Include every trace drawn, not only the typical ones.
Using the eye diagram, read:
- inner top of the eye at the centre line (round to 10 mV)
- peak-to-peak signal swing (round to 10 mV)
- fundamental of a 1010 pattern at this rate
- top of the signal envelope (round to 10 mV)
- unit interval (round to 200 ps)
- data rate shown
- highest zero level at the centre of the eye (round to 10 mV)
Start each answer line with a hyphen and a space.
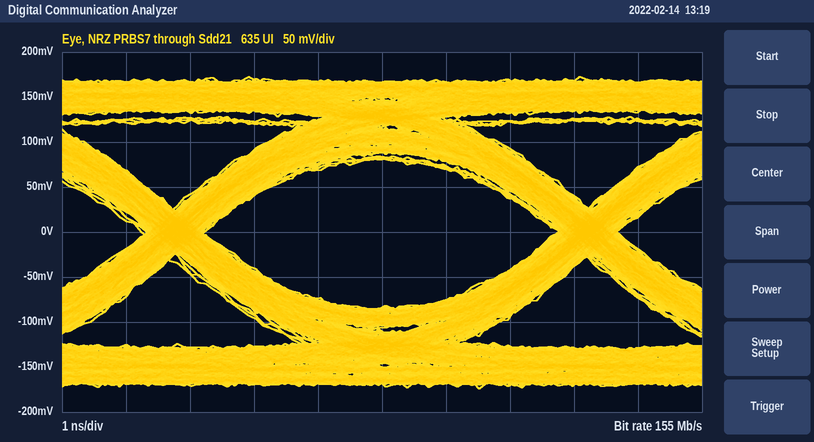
- 80 mV
- 350 mV
- 77.5 MHz
- 170 mV
- 6.4 ns
- 155 Mb/s
- -80 mV
